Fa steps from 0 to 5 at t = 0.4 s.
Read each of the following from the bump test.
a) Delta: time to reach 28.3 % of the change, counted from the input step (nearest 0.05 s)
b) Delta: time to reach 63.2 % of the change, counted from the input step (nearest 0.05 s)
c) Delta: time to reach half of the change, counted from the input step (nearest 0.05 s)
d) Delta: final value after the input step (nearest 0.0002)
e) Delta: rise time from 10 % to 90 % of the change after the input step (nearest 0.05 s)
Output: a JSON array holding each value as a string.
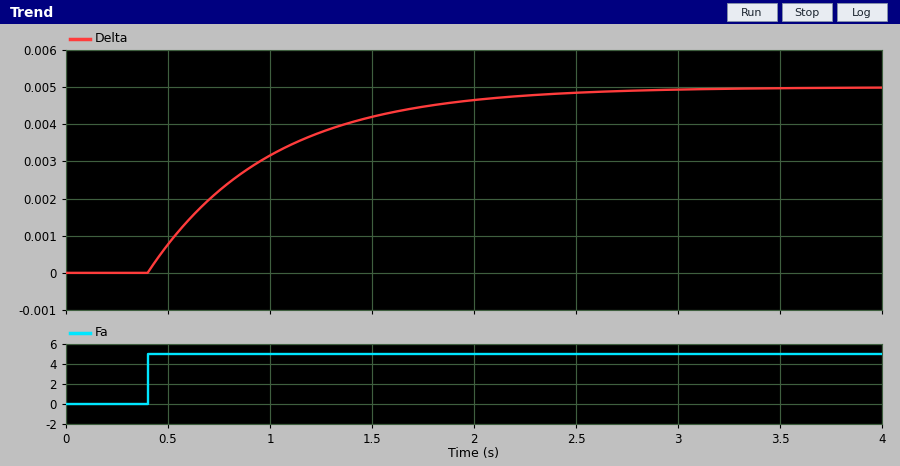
["0.20 s", "0.60 s", "0.40 s", "0.0050", "1.30 s"]
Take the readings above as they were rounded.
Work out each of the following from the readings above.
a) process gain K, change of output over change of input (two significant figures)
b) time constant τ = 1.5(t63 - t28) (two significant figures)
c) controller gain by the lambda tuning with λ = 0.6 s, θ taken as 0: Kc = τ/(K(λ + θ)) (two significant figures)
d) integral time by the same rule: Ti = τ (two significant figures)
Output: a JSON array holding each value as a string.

["0.0010", "0.60 s", "1000", "0.60 s"]
